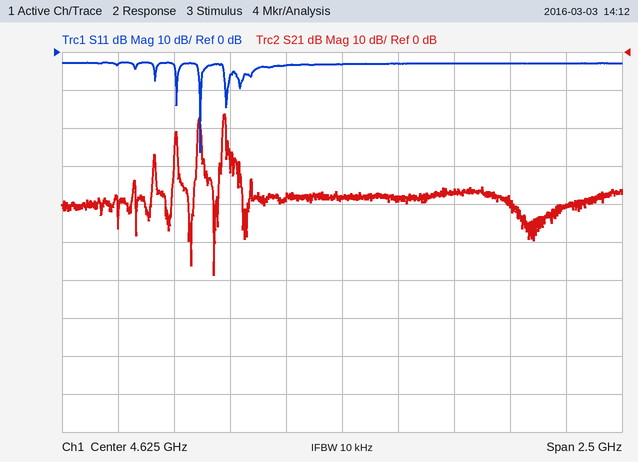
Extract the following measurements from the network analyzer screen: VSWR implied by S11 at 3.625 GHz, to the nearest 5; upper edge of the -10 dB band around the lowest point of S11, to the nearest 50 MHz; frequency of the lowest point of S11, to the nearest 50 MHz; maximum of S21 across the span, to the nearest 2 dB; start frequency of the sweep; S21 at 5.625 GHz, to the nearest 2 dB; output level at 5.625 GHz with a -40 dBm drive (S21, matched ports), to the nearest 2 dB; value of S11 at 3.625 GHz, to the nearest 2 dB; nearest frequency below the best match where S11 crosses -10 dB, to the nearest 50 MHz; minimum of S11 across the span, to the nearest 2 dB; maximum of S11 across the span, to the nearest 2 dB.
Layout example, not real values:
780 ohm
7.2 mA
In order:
5
4.00 GHz
4.00 GHz
-16 dB
3.375 GHz
-40 dB
-80 dBm
-4 dB
4.00 GHz
-26 dB
-2 dB
